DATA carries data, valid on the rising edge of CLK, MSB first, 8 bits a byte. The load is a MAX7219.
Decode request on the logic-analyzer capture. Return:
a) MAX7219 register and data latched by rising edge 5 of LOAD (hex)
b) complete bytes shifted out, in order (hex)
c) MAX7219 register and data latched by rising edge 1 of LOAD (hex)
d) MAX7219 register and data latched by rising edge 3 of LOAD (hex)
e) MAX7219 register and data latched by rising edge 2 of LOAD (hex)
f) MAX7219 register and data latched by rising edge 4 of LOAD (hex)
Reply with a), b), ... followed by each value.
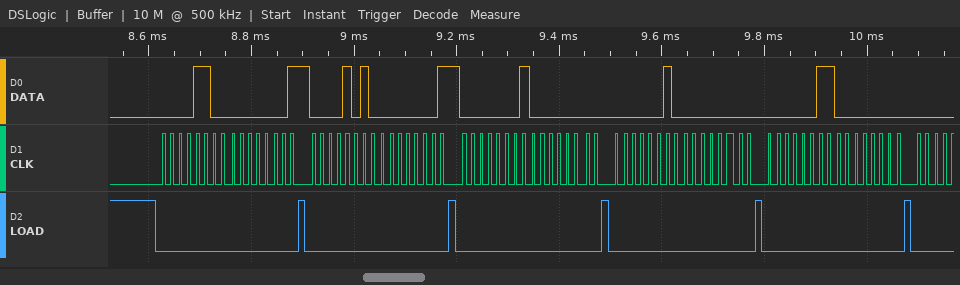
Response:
a) register 0x3, data 0x00
b) 0x0C 0x01 0x0A 0x01 0x01 0x00 0x02 0x00 0x03 0x00
c) register 0xC, data 0x01
d) register 0x1, data 0x00
e) register 0xA, data 0x01
f) register 0x2, data 0x00
